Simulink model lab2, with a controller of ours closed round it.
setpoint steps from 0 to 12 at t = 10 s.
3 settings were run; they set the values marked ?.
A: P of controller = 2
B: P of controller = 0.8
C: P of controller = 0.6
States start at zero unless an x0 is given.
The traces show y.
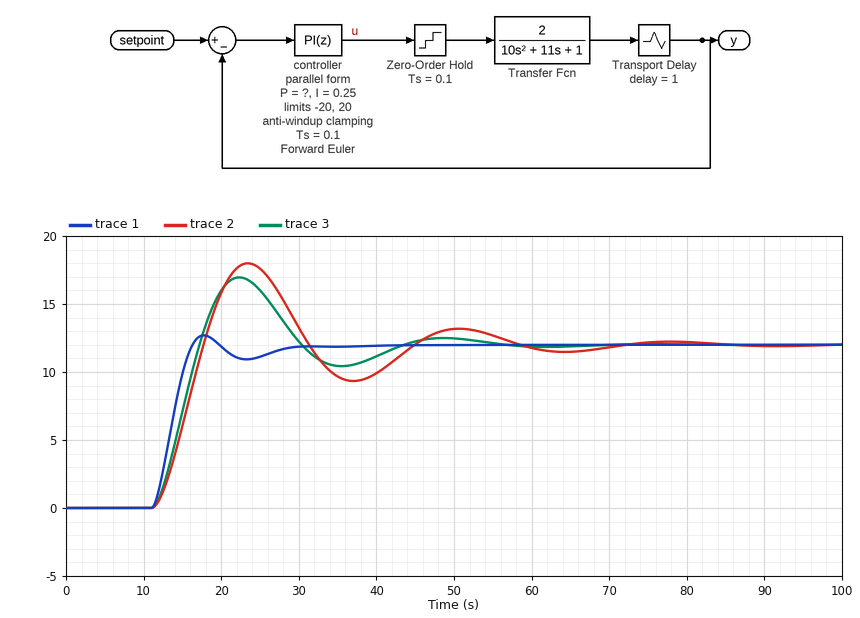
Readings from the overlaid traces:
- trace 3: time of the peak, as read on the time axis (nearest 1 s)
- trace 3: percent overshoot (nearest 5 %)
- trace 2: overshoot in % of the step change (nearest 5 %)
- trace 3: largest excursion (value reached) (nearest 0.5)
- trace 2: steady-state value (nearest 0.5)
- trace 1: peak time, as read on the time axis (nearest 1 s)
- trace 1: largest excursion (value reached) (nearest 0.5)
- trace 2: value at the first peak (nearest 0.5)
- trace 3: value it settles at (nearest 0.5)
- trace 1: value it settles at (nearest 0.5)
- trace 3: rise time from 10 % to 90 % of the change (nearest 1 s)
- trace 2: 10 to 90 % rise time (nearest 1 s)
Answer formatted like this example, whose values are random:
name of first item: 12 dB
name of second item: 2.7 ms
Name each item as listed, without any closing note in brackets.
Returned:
trace 3: time of the peak, as read on the time axis: 22 s
trace 3: percent overshoot: 40 %
trace 2: overshoot in % of the step change: 50 %
trace 3: largest excursion (value reached): 17.0
trace 2: steady-state value: 12.0
trace 1: peak time, as read on the time axis: 18 s
trace 1: largest excursion (value reached): 12.5
trace 2: value at the first peak: 18.0
trace 3: value it settles at: 12.0
trace 1: value it settles at: 12.0
trace 3: rise time from 10 % to 90 % of the change: 4 s
trace 2: 10 to 90 % rise time: 5 s
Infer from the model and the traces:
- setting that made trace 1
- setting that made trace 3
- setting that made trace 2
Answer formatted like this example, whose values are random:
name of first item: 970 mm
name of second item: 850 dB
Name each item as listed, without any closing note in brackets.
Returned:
setting that made trace 1: A
setting that made trace 3: B
setting that made trace 2: C
